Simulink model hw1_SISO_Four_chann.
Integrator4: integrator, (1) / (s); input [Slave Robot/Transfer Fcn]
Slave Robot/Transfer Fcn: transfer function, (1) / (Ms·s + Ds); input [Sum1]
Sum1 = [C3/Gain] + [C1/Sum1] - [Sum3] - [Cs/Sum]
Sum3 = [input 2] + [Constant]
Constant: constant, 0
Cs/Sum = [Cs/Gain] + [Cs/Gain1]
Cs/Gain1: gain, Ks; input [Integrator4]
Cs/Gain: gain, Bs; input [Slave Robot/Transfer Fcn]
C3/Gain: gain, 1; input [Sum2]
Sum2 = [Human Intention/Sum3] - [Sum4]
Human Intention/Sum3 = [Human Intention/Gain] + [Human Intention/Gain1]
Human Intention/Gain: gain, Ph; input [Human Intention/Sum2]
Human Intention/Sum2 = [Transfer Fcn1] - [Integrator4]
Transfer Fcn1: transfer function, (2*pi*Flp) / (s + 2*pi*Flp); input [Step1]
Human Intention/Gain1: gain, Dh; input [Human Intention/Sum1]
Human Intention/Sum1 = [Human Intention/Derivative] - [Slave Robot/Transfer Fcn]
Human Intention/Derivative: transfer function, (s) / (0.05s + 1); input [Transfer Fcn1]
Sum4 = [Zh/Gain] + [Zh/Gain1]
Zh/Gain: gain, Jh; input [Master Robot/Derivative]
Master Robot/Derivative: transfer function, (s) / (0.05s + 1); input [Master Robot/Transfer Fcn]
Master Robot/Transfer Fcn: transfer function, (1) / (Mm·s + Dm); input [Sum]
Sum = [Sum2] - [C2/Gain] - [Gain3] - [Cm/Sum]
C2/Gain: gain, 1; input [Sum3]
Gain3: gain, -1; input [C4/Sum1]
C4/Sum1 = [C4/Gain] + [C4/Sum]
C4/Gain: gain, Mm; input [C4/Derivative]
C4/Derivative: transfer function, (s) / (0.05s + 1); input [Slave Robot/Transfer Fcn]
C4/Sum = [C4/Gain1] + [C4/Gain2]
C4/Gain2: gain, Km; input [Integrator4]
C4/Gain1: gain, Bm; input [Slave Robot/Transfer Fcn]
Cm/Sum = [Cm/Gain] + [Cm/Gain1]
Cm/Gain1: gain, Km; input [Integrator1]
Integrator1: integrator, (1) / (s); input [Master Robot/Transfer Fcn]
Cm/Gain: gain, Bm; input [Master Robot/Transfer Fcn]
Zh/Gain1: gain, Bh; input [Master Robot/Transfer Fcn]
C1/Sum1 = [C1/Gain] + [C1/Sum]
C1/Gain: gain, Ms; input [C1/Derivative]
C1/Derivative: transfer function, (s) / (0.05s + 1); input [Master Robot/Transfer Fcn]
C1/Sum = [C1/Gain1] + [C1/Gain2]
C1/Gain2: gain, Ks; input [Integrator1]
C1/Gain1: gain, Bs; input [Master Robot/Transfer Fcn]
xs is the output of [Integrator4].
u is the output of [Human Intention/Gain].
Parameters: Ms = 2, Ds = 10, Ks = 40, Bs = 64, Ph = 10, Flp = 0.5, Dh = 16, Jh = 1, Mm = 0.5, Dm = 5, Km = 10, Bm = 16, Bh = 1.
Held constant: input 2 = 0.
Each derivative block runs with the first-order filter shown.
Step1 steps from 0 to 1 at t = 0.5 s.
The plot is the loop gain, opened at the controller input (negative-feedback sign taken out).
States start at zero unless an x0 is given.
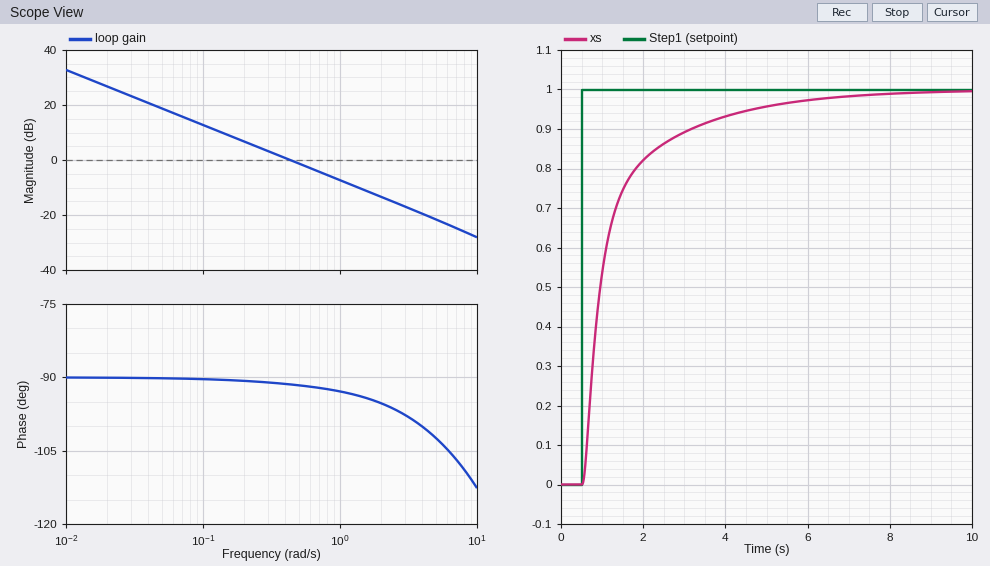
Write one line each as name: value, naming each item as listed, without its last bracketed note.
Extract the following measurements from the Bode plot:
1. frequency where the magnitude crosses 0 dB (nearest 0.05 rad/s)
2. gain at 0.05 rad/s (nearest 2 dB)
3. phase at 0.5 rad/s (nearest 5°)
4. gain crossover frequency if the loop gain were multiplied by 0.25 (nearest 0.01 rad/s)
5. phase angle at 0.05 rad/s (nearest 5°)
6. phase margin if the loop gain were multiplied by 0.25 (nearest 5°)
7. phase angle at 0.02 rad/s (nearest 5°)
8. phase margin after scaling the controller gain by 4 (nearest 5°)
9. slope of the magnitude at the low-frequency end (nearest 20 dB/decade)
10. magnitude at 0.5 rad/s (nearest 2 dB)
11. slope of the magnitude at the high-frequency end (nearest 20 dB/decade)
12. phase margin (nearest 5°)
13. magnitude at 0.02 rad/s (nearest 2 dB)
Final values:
frequency where the magnitude crosses 0 dB: 0.45 rad/s
gain at 0.05 rad/s: 18 dB
phase at 0.5 rad/s: -90°
gain crossover frequency if the loop gain were multiplied by 0.25: 0.11 rad/s
phase angle at 0.05 rad/s: -90°
phase margin if the loop gain were multiplied by 0.25: 90°
phase angle at 0.02 rad/s: -90°
phase margin after scaling the controller gain by 4: 85°
slope of the magnitude at the low-frequency end: -20 dB/decade
magnitude at 0.5 rad/s: -2 dB
slope of the magnitude at the high-frequency end: -20 dB/decade
phase margin: 90°
magnitude at 0.02 rad/s: 26 dB
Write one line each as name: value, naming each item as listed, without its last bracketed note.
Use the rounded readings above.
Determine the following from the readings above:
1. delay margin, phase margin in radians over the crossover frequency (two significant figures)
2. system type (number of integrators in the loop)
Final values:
delay margin, phase margin in radians over the crossover frequency: 3.5 s
system type: 1
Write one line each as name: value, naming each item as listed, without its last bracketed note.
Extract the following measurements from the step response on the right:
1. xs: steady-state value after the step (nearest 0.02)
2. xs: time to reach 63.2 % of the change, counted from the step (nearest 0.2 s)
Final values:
xs: steady-state value after the step: 1.00
xs: time to reach 63.2 % of the change, counted from the step: 0.6 s
